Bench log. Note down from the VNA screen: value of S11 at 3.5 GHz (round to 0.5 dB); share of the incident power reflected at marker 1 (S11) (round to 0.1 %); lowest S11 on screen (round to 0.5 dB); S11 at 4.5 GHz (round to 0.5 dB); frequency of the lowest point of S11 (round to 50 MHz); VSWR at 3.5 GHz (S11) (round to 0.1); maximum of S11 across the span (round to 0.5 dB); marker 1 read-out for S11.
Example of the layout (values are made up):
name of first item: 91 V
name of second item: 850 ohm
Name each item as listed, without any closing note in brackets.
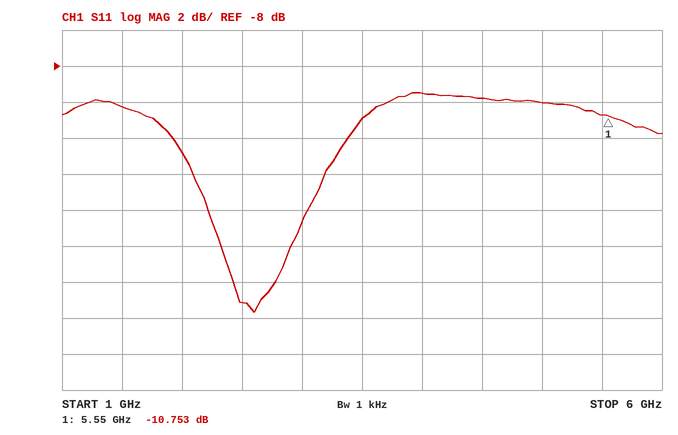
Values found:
value of S11 at 3.5 GHz: -11.0 dB
share of the incident power reflected at marker 1 (S11): 8.4 %
lowest S11 on screen: -21.5 dB
S11 at 4.5 GHz: -10.0 dB
frequency of the lowest point of S11: 2.60 GHz
VSWR at 3.5 GHz (S11): 1.8
maximum of S11 across the span: -9.5 dB
marker 1 read-out for S11: -10.753 dB
